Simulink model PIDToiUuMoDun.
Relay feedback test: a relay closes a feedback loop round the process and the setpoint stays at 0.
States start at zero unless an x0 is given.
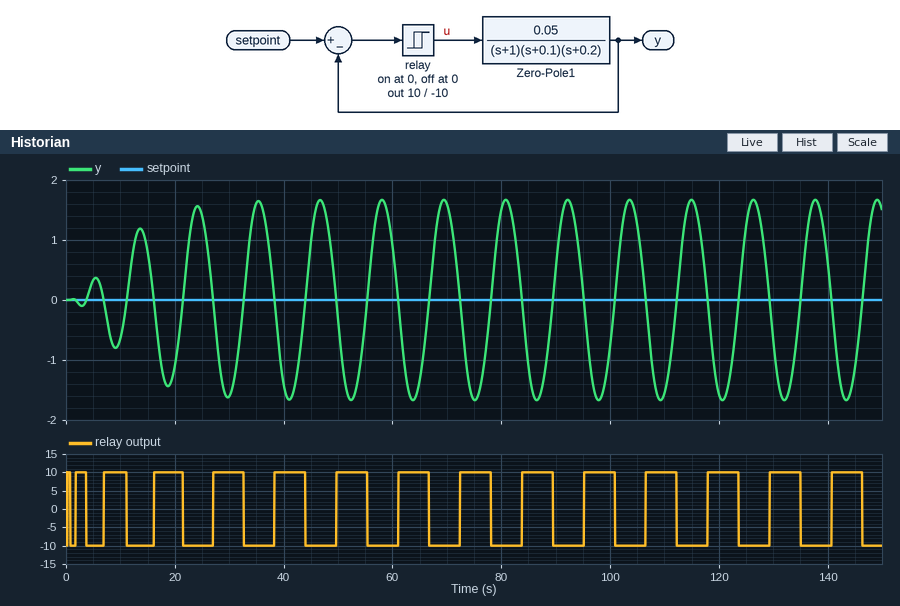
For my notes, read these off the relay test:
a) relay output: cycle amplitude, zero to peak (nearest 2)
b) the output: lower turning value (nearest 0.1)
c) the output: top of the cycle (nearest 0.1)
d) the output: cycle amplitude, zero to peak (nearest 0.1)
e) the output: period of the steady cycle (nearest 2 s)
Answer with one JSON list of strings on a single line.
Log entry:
["10", "-1.7", "1.7", "1.7", "12 s"]
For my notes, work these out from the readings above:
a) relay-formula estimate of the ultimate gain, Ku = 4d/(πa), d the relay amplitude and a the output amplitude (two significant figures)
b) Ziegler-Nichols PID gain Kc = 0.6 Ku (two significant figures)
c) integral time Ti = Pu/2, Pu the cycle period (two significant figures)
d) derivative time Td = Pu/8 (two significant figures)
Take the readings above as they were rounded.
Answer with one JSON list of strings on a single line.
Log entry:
["7.5", "4.5", "6.0 s", "1.5 s"]
